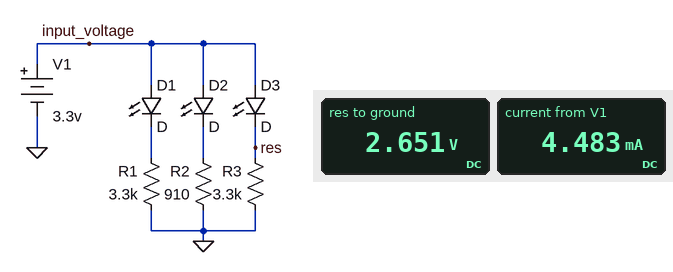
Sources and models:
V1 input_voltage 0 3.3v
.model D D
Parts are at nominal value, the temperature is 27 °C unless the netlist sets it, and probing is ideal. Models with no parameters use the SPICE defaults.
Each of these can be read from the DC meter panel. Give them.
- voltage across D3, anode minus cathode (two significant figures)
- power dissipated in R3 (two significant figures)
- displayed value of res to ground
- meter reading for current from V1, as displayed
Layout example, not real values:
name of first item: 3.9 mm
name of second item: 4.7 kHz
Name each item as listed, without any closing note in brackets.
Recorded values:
voltage across D3, anode minus cathode: 650 mV
power dissipated in R3: 2.1 mW
displayed value of res to ground: 2.651 V
meter reading for current from V1, as displayed: 4.483 mA
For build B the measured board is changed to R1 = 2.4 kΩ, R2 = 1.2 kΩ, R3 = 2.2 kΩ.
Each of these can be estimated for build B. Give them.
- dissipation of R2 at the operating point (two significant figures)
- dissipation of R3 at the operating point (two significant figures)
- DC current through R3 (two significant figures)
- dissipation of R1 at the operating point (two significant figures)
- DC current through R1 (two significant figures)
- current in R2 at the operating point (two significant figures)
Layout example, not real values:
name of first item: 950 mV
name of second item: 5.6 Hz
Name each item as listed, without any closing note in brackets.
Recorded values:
dissipation of R2 at the operating point: 5.7 mW
dissipation of R3 at the operating point: 3.2 mW
DC current through R3: 1.2 mA
dissipation of R1 at the operating point: 2.9 mW
DC current through R1: 1.1 mA
current in R2 at the operating point: 2.2 mA
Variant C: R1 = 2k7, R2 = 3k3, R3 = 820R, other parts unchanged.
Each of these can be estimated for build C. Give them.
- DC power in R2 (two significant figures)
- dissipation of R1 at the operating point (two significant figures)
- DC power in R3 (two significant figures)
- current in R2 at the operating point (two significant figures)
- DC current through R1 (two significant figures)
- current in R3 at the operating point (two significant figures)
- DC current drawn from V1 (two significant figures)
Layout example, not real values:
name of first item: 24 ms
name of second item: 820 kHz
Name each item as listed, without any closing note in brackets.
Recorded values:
DC power in R2: 2.1 mW
dissipation of R1 at the operating point: 2.6 mW
DC power in R3: 8.3 mW
current in R2 at the operating point: 800 µA
DC current through R1: 980 µA
current in R3 at the operating point: 3.2 mA
DC current drawn from V1: 5.0 mA
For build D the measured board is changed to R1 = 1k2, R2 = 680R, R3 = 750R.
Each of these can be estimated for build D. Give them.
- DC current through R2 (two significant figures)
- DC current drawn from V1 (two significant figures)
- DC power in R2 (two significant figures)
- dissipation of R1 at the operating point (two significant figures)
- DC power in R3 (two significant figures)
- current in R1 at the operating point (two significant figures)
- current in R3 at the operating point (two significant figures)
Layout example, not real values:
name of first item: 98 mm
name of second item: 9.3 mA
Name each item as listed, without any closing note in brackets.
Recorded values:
DC current through R2: 3.8 mA
DC current drawn from V1: 9.5 mA
DC power in R2: 10 mW
dissipation of R1 at the operating point: 5.7 mW
DC power in R3: 9.1 mW
current in R1 at the operating point: 2.2 mA
current in R3 at the operating point: 3.5 mA
